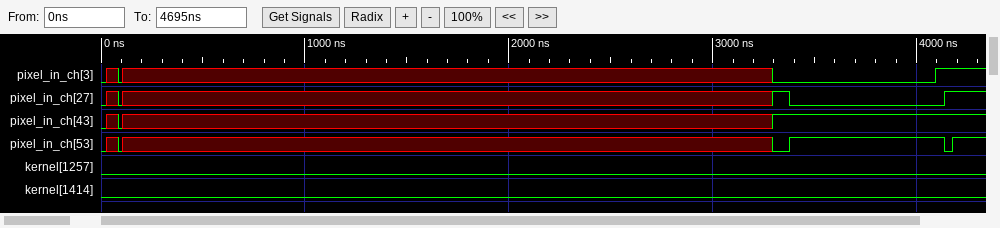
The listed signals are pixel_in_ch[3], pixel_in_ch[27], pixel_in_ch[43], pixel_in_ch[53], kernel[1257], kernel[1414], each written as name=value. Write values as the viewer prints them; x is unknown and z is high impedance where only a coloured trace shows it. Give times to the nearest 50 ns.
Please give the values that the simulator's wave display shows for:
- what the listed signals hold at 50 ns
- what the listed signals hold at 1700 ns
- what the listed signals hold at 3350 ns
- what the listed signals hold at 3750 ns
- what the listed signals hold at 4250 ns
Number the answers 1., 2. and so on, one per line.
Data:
1. pixel_in_ch[3]=x, pixel_in_ch[27]=x, pixel_in_ch[43]=x, pixel_in_ch[53]=x, kernel[1257]=0, kernel[1414]=0
2. pixel_in_ch[3]=x, pixel_in_ch[27]=x, pixel_in_ch[43]=x, pixel_in_ch[53]=x, kernel[1257]=0, kernel[1414]=0
3. pixel_in_ch[3]=0, pixel_in_ch[27]=1, pixel_in_ch[43]=1, pixel_in_ch[53]=0, kernel[1257]=0, kernel[1414]=0
4. pixel_in_ch[3]=0, pixel_in_ch[27]=0, pixel_in_ch[43]=1, pixel_in_ch[53]=1, kernel[1257]=0, kernel[1414]=0
5. pixel_in_ch[3]=1, pixel_in_ch[27]=1, pixel_in_ch[43]=1, pixel_in_ch[53]=1, kernel[1257]=0, kernel[1414]=0
